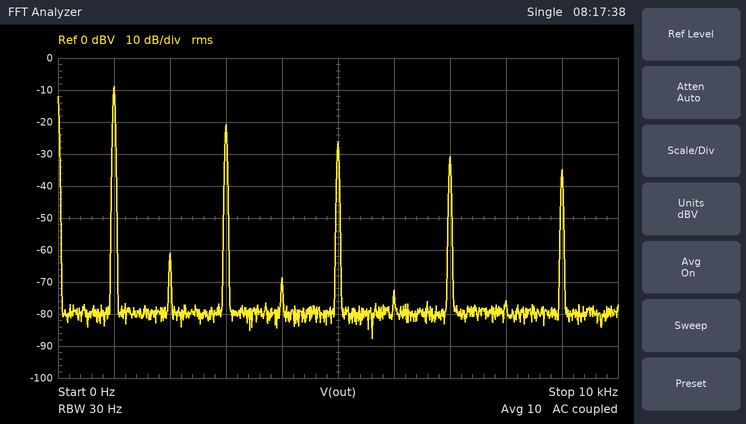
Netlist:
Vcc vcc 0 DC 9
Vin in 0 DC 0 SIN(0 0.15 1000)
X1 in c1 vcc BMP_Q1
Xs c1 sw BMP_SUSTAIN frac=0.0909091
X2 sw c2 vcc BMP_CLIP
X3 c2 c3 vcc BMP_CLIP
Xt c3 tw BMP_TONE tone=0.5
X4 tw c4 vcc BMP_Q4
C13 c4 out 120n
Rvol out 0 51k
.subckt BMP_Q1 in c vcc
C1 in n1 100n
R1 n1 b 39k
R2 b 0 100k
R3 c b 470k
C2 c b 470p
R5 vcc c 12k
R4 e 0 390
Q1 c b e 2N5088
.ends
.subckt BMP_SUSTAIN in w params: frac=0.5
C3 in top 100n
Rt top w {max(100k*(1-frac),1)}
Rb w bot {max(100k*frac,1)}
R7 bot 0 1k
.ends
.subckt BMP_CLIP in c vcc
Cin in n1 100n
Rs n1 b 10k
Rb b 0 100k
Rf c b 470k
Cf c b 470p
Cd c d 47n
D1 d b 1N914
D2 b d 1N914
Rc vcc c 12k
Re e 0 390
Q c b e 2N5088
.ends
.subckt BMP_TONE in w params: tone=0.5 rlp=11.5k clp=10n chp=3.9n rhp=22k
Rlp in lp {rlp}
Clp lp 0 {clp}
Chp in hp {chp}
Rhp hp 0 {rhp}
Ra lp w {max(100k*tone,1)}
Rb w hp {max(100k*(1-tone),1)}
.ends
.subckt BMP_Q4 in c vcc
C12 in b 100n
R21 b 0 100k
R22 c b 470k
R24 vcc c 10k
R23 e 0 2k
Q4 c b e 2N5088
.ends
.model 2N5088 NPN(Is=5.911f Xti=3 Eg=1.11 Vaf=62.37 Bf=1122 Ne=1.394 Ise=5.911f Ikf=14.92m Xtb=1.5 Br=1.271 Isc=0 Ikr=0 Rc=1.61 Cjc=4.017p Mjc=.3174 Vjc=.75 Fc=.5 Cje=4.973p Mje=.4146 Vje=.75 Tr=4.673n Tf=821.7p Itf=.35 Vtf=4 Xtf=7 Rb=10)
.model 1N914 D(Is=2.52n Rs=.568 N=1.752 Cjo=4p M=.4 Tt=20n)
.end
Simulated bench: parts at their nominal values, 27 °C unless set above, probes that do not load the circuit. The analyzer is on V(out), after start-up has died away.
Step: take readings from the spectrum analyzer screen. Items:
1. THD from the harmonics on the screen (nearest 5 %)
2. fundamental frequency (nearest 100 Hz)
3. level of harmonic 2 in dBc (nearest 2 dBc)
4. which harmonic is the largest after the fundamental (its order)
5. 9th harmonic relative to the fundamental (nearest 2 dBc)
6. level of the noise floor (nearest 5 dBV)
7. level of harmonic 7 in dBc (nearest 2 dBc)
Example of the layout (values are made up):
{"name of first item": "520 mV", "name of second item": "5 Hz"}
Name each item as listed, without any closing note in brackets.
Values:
{"THD from the harmonics on the screen": "30 %", "fundamental frequency": "1.0 kHz", "level of harmonic 2 in dBc": "-52 dBc", "which harmonic is the largest after the fundamental": "3", "9th harmonic relative to the fundamental": "-26 dBc", "level of the noise floor": "-80 dBV", "level of harmonic 7 in dBc": "-22 dBc"}
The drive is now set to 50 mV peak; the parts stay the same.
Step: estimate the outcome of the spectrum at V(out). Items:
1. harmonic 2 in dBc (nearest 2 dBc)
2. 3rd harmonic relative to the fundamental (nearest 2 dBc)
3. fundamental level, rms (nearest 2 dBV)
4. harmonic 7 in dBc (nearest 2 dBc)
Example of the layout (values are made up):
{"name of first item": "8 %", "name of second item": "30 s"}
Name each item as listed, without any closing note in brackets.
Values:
{"harmonic 2 in dBc": "-54 dBc", "3rd harmonic relative to the fundamental": "-14 dBc", "fundamental level, rms": "-10 dBV", "harmonic 7 in dBc": "-28 dBc"}
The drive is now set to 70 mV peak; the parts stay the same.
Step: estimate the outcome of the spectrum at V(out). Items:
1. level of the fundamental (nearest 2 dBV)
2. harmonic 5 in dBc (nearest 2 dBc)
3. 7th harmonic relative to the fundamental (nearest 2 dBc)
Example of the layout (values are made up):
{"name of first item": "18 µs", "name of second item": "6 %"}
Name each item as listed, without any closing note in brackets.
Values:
{"level of the fundamental": "-10 dBV", "harmonic 5 in dBc": "-20 dBc", "7th harmonic relative to the fundamental": "-26 dBc"}
